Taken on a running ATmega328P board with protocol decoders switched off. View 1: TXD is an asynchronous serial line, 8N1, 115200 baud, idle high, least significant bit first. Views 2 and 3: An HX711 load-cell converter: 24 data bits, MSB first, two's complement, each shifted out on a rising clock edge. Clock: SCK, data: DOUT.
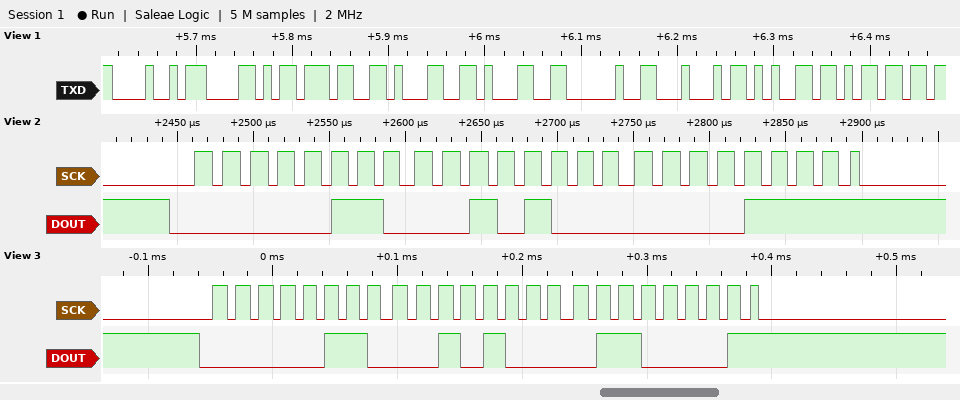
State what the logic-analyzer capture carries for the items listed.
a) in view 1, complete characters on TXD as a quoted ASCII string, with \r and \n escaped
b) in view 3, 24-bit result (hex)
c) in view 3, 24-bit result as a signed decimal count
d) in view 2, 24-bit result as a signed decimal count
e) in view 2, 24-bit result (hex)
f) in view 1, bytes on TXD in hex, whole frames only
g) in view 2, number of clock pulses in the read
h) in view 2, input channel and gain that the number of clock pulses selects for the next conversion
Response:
"HX711 Dem"
0x062861
403553
403471
0x06280F
48 58 37 31 31 20 44 65 6D
25
channel A, gain 128
